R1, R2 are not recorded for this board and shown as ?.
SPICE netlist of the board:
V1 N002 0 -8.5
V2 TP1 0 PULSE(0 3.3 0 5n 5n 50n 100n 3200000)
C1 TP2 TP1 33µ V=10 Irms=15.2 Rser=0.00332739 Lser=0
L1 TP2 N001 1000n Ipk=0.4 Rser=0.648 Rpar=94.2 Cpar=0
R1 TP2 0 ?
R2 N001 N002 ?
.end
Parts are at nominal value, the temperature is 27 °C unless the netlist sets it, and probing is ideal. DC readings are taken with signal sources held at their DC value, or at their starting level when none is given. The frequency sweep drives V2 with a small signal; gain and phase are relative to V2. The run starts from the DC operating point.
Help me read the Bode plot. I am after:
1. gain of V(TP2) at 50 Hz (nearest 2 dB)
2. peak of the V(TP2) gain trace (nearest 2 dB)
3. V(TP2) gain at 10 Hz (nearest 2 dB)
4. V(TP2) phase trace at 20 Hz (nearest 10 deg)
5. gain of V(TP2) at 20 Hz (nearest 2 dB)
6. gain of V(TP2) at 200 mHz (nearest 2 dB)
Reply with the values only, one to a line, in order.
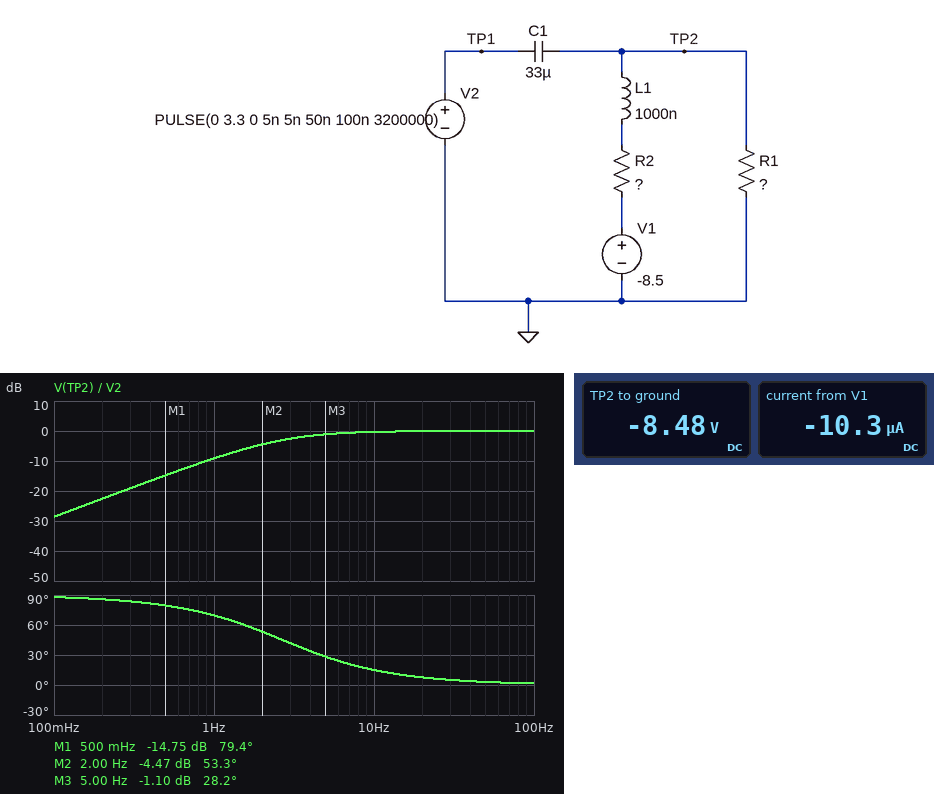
0 dB
0 dB
0 dB
10 deg
0 dB
-22 dB
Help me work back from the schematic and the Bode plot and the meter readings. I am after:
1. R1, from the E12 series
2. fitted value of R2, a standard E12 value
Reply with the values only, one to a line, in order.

820 kΩ
1.8 kΩ
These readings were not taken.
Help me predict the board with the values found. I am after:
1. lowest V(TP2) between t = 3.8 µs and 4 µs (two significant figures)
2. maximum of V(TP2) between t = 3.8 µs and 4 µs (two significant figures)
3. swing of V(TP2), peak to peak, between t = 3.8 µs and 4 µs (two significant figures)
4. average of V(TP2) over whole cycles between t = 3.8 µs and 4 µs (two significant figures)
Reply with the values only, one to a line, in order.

-8.5 V
-5.2 V
3.3 V
-6.7 V
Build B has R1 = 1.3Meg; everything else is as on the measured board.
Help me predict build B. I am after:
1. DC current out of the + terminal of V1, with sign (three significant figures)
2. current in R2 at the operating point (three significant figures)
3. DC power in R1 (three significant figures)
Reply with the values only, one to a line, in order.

-6.53 µA
6.53 µA
55.4 µW
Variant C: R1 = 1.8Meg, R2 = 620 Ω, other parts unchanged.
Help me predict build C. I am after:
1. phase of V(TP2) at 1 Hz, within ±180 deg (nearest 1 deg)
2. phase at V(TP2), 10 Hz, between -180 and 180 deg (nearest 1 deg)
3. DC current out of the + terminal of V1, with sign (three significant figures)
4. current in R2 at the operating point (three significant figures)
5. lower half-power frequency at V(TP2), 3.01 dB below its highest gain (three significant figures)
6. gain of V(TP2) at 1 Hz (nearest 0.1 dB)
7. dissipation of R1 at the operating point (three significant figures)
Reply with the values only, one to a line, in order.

83 deg
38 deg
-4.72 µA
4.72 µA
7.77 Hz
-17.9 dB
40.1 µW
